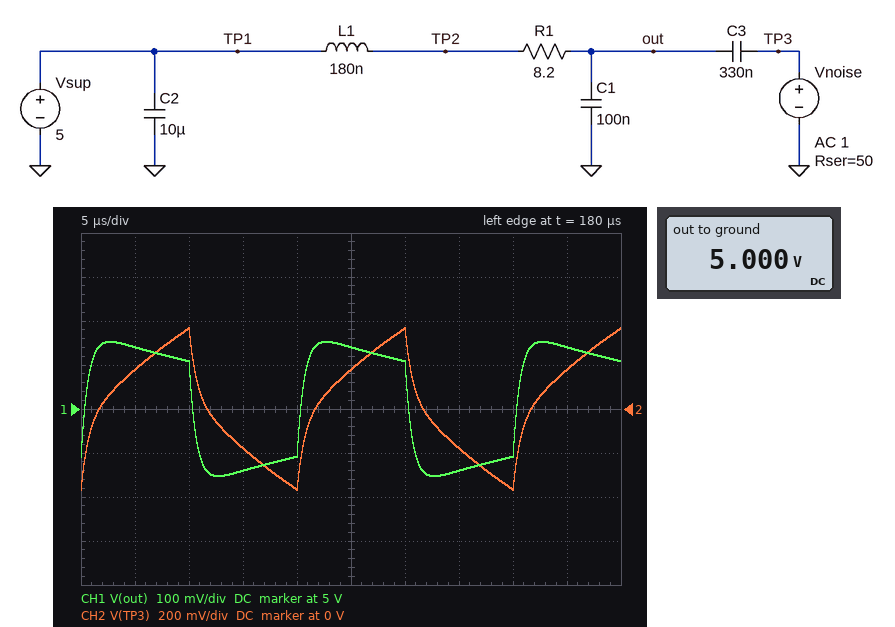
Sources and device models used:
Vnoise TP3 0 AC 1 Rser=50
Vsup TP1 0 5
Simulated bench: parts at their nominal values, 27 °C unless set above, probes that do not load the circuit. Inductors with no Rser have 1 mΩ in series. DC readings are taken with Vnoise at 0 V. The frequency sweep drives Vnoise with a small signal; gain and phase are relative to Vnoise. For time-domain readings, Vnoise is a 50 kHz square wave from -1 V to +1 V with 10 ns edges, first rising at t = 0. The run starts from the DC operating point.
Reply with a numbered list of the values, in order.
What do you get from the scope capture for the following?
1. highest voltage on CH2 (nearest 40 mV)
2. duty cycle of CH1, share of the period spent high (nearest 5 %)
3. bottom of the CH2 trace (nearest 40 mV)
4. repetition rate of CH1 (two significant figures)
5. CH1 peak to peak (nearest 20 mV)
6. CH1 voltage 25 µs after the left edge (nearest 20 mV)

1. 360 mV
2. 50 %
3. -360 mV
4. 50 kHz
5. 300 mV
6. 5.14 V
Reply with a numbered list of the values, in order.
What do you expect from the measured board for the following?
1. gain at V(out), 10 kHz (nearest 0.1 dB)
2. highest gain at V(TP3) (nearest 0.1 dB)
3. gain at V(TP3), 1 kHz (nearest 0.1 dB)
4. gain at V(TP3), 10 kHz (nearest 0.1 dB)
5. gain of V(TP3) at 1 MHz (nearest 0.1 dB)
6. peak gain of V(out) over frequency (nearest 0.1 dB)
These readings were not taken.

1. -19.3 dB
2. 0 dB
3. -0.1 dB
4. -3.7 dB
5. -27.7 dB
6. -17.4 dB
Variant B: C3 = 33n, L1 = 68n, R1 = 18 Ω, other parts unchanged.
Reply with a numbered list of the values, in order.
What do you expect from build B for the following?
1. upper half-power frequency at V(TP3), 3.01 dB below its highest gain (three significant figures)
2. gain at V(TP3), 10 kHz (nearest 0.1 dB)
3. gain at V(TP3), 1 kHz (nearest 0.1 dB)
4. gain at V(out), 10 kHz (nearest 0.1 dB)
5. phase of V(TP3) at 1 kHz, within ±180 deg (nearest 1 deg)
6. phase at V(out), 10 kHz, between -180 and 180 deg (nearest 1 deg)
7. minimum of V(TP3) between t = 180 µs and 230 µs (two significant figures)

1. 101 kHz
2. -0.1 dB
3. 0 dB
4. -28.7 dB
5. -1 deg
6. 76 deg
7. -980 mV
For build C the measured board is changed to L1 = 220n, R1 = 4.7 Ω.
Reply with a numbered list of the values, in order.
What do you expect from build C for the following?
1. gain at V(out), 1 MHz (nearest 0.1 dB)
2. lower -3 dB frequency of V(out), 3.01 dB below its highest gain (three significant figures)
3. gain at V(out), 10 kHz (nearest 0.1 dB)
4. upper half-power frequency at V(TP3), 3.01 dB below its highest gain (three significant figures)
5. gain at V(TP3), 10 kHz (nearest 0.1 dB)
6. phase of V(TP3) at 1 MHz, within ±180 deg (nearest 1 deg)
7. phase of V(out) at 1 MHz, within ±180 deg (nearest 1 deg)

1. -29.7 dB
2. 8.45 kHz
3. -23.8 dB
4. 8.90 kHz
5. -3.5 dB
6. -73 deg
7. -69 deg
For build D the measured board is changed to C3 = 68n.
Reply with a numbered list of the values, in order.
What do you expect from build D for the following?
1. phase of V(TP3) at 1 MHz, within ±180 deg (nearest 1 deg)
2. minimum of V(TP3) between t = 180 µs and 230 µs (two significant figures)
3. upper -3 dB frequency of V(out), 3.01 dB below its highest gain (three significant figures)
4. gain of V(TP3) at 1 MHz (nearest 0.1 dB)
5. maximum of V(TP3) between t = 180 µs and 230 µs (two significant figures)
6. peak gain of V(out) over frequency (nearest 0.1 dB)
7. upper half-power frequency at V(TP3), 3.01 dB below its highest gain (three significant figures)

1. -81 deg
2. -870 mV
3. 309 kHz
4. -22.2 dB
5. 870 mV
6. -18.6 dB
7. 42.5 kHz
